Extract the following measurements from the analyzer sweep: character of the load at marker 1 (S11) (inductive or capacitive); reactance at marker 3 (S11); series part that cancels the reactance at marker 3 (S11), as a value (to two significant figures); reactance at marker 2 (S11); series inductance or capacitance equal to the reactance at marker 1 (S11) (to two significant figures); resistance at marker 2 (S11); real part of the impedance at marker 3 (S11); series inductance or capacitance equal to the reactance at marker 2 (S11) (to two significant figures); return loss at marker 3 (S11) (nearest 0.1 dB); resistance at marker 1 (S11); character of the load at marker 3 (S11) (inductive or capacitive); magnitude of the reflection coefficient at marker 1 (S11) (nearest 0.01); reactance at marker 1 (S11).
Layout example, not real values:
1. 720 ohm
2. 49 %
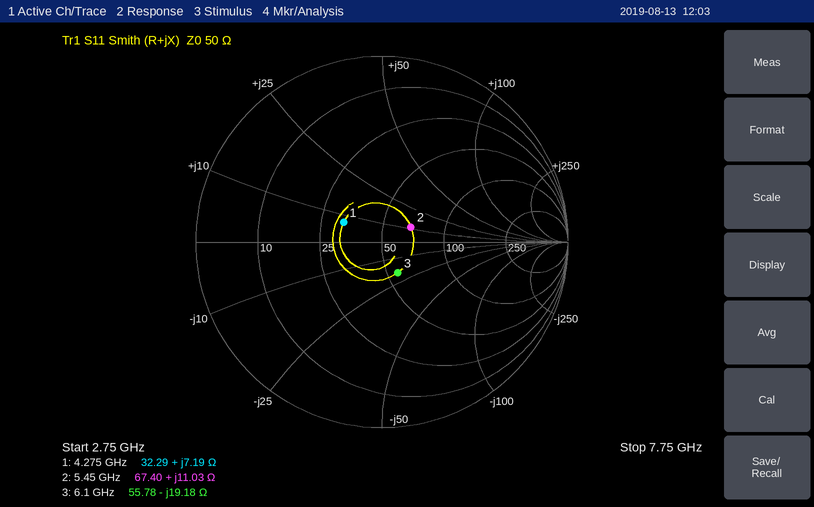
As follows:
1. inductive
2. -19.18 Ω
3. 500 pH
4. +11.03 Ω
5. 270 pH
6. 67.40 Ω
7. 55.78 Ω
8. 320 pH
9. 14.6 dB
10. 32.29 Ω
11. capacitive
12. 0.23
13. +7.19 Ω
